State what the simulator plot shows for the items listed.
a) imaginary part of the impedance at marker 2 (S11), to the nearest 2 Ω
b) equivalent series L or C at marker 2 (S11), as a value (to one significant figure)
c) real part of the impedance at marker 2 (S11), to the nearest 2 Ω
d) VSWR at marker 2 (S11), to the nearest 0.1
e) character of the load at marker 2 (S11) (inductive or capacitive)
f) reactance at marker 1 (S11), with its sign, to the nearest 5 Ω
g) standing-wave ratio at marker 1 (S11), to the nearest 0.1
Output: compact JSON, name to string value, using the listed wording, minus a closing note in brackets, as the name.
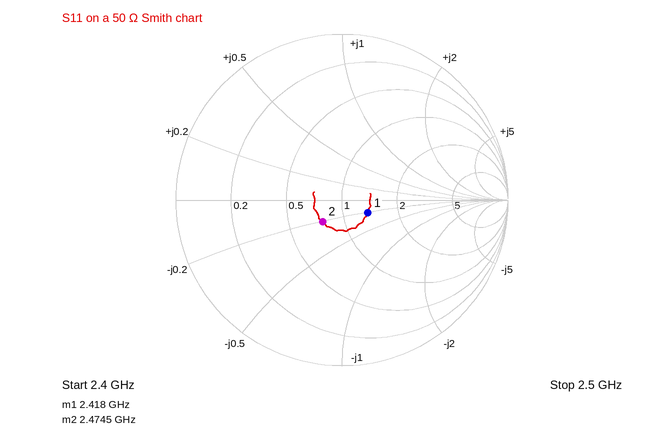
{"imaginary part of the impedance at marker 2 (S11), to the nearest 2 Ω": "-10 Ω", "equivalent series L or C at marker 2 (S11), as a value": "6 pF", "real part of the impedance at marker 2 (S11), to the nearest 2 Ω": "38 Ω", "VSWR at marker 2 (S11), to the nearest 0.1": "1.4", "character of the load at marker 2 (S11)": "capacitive", "reactance at marker 1 (S11), with its sign, to the nearest 5 Ω": "-10 Ω", "standing-wave ratio at marker 1 (S11), to the nearest 0.1": "1.4"}
